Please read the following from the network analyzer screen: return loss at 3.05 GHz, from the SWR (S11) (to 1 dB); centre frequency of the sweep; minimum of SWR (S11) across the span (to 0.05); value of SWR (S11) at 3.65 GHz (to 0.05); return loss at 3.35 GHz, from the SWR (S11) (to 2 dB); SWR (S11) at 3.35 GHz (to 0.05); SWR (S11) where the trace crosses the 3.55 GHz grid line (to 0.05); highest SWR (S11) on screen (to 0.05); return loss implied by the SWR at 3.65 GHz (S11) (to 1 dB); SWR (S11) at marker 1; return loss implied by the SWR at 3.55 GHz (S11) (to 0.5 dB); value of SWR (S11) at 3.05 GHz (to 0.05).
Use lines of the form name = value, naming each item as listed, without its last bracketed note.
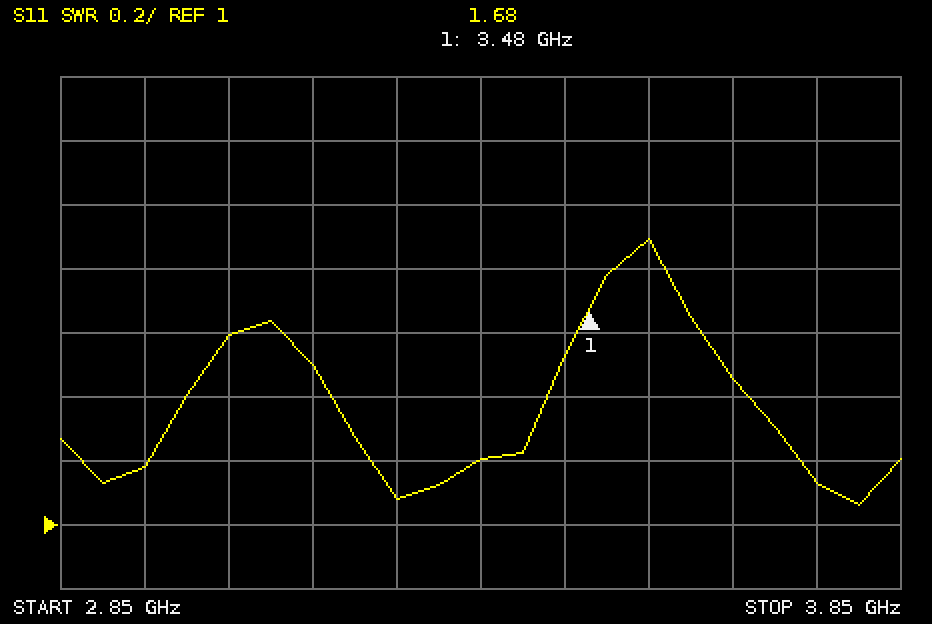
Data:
return loss at 3.05 GHz, from the SWR (S11) = 13 dB
centre frequency of the sweep = 3.35 GHz
minimum of SWR (S11) across the span = 1.05
value of SWR (S11) at 3.65 GHz = 1.45
return loss at 3.35 GHz, from the SWR (S11) = 20 dB
SWR (S11) at 3.35 GHz = 1.20
SWR (S11) where the trace crosses the 3.55 GHz grid line = 1.90
highest SWR (S11) on screen = 1.90
return loss implied by the SWR at 3.65 GHz (S11) = 15 dB
SWR (S11) at marker 1 = 1.68
return loss implied by the SWR at 3.55 GHz (S11) = 10.0 dB
value of SWR (S11) at 3.05 GHz = 1.60
